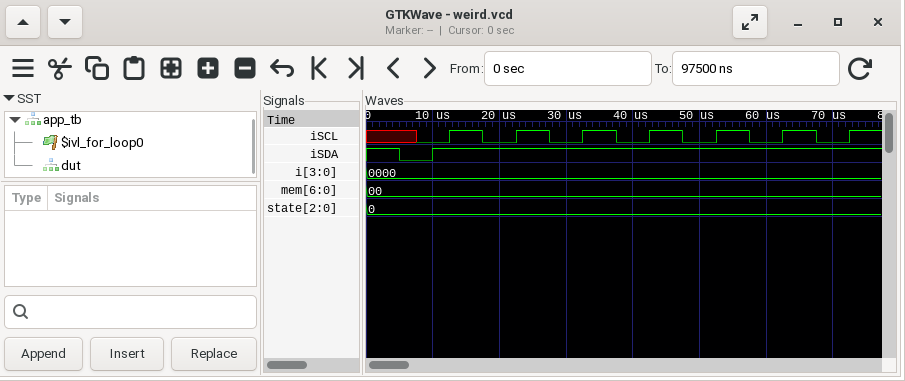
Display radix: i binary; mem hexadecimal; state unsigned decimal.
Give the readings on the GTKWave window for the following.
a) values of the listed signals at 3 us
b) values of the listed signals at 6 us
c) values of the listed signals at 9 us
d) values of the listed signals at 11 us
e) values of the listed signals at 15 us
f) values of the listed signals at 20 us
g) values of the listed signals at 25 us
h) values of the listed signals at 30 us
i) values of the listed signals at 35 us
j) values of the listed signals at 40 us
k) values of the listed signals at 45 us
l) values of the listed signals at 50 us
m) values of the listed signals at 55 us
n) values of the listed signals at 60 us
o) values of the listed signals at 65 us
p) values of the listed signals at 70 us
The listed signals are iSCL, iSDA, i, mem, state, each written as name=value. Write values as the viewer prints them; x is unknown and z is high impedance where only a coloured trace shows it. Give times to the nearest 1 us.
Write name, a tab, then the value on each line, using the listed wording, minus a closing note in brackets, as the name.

values of the listed signals at 3 us	iSCL=x, iSDA=1, i=0000, mem=00, state=0
values of the listed signals at 6 us	iSCL=x, iSDA=0, i=0000, mem=00, state=0
values of the listed signals at 9 us	iSCL=0, iSDA=0, i=0000, mem=00, state=0
values of the listed signals at 11 us	iSCL=0, iSDA=1, i=0000, mem=00, state=0
values of the listed signals at 15 us	iSCL=1, iSDA=1, i=0000, mem=00, state=0
values of the listed signals at 20 us	iSCL=0, iSDA=1, i=0000, mem=00, state=0
values of the listed signals at 25 us	iSCL=1, iSDA=1, i=0000, mem=00, state=0
values of the listed signals at 30 us	iSCL=0, iSDA=1, i=0000, mem=00, state=0
values of the listed signals at 35 us	iSCL=1, iSDA=1, i=0000, mem=00, state=0
values of the listed signals at 40 us	iSCL=0, iSDA=1, i=0000, mem=00, state=0
values of the listed signals at 45 us	iSCL=1, iSDA=1, i=0000, mem=00, state=0
values of the listed signals at 50 us	iSCL=0, iSDA=1, i=0000, mem=00, state=0
values of the listed signals at 55 us	iSCL=1, iSDA=1, i=0000, mem=00, state=0
values of the listed signals at 60 us	iSCL=0, iSDA=1, i=0000, mem=00, state=0
values of the listed signals at 65 us	iSCL=1, iSDA=1, i=0000, mem=00, state=0
values of the listed signals at 70 us	iSCL=0, iSDA=1, i=0000, mem=00, state=0
